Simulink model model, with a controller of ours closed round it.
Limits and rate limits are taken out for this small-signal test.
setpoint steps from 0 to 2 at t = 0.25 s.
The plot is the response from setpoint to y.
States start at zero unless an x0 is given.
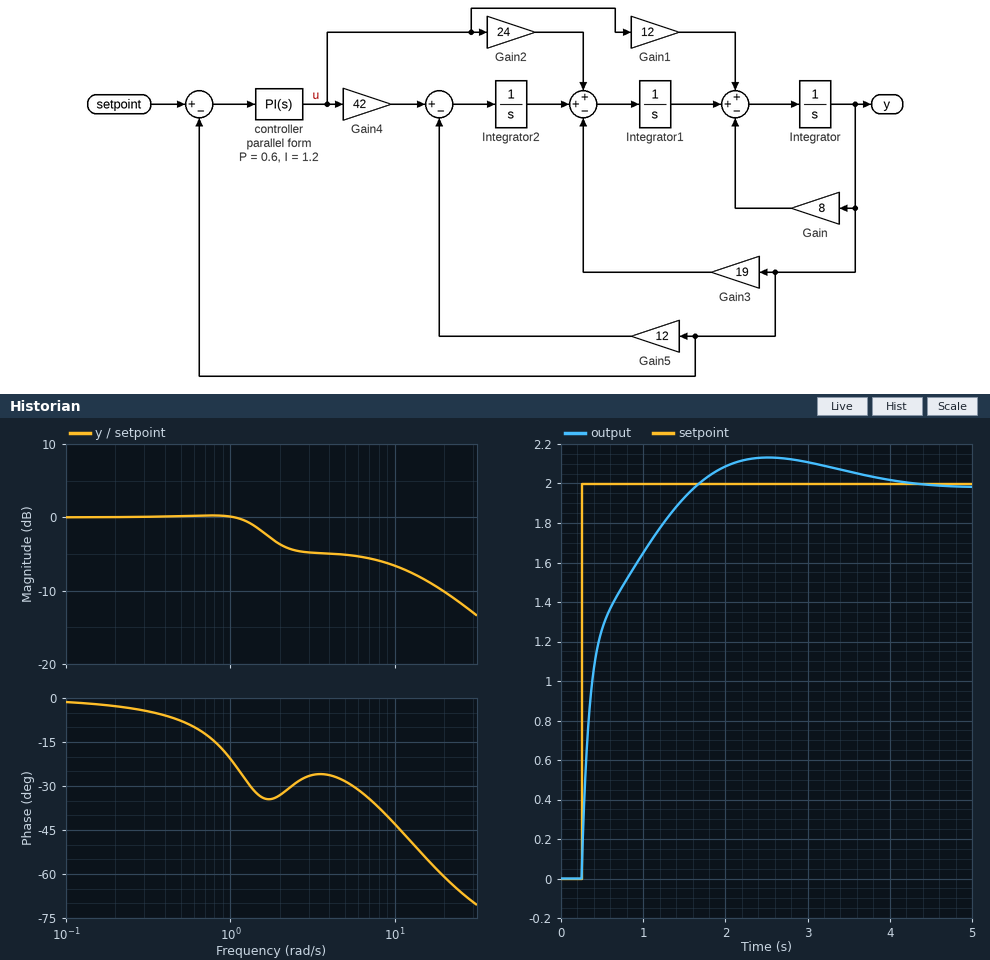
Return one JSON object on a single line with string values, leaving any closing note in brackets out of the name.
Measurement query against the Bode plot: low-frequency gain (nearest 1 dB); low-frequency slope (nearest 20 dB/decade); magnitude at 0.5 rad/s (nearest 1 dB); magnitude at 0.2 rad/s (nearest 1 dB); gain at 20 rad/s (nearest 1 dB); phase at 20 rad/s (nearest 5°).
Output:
{"low-frequency gain": "0 dB", "low-frequency slope": "0 dB/decade", "magnitude at 0.5 rad/s": "0 dB", "magnitude at 0.2 rad/s": "0 dB", "gain at 20 rad/s": "-10 dB", "phase at 20 rad/s": "-60°"}
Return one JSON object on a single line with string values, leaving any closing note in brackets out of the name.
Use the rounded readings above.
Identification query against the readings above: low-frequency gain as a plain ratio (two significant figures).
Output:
{"low-frequency gain as a plain ratio": "1.0"}
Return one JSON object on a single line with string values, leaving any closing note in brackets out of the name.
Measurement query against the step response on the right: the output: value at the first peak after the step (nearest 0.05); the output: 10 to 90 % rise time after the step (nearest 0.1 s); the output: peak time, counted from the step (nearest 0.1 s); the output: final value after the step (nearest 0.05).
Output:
{"the output: value at the first peak after the step": "2.15", "the output: 10 to 90 % rise time after the step": "1.0 s", "the output: peak time, counted from the step": "2.3 s", "the output: final value after the step": "2.00"}
